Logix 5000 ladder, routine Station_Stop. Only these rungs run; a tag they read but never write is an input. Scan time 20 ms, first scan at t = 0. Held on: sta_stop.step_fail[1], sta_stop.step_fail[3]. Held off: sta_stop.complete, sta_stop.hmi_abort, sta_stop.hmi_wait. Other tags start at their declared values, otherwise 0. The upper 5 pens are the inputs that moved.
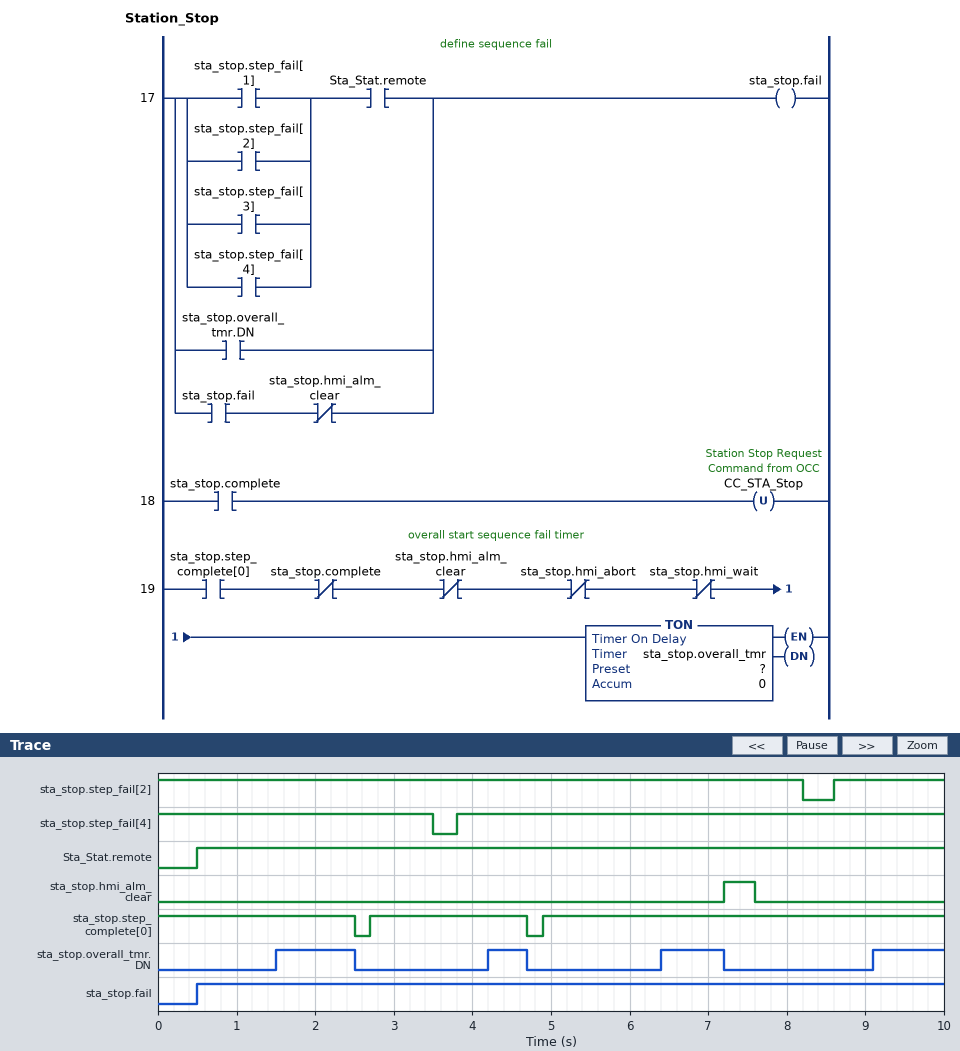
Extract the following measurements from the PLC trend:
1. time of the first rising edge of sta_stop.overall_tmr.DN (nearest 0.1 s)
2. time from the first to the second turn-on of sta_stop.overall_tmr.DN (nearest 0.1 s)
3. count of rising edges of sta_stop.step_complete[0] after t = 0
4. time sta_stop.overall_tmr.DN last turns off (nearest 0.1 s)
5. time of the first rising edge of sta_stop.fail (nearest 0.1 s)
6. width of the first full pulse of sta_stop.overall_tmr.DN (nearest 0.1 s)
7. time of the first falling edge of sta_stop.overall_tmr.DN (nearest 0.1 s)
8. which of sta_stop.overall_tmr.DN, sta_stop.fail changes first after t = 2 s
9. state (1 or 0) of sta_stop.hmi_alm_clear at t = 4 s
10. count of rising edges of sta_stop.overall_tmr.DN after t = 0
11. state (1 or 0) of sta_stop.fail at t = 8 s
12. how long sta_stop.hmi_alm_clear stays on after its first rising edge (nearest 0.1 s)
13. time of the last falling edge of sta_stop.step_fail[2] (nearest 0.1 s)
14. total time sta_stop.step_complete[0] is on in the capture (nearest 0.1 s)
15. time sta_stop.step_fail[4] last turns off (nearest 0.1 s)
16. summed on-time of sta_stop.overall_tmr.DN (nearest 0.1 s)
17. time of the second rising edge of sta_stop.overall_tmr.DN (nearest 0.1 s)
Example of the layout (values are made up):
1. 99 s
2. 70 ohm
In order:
1. 1.5 s
2. 2.7 s
3. 2
4. 7.2 s
5. 0.5 s
6. 1.0 s
7. 2.5 s
8. sta_stop.overall_tmr.DN
9. 0
10. 4
11. 1
12. 0.4 s
13. 8.2 s
14. 9.6 s
15. 3.5 s
16. 3.2 s
17. 4.2 s
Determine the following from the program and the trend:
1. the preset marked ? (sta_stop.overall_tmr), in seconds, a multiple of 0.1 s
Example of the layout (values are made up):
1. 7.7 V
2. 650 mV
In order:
1. 1.5 s
